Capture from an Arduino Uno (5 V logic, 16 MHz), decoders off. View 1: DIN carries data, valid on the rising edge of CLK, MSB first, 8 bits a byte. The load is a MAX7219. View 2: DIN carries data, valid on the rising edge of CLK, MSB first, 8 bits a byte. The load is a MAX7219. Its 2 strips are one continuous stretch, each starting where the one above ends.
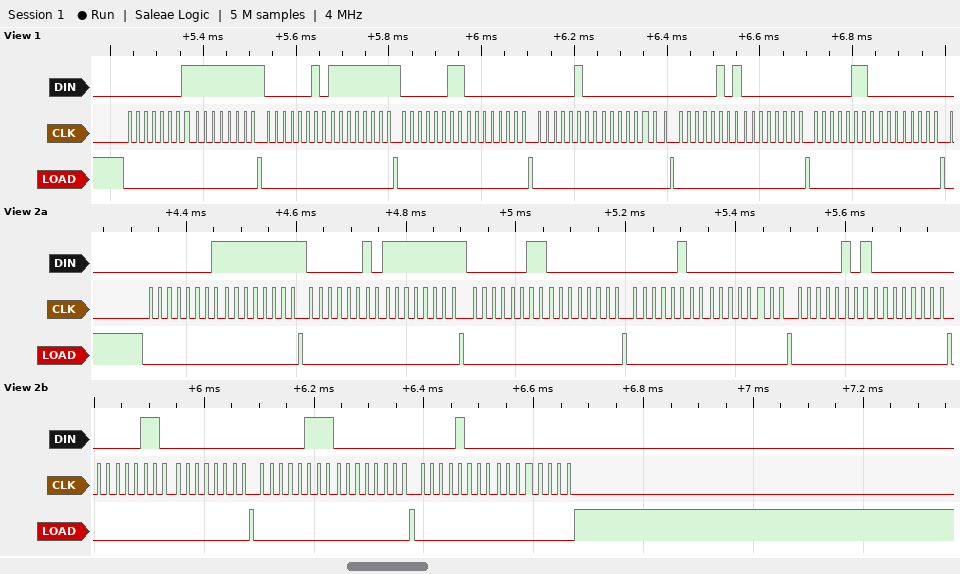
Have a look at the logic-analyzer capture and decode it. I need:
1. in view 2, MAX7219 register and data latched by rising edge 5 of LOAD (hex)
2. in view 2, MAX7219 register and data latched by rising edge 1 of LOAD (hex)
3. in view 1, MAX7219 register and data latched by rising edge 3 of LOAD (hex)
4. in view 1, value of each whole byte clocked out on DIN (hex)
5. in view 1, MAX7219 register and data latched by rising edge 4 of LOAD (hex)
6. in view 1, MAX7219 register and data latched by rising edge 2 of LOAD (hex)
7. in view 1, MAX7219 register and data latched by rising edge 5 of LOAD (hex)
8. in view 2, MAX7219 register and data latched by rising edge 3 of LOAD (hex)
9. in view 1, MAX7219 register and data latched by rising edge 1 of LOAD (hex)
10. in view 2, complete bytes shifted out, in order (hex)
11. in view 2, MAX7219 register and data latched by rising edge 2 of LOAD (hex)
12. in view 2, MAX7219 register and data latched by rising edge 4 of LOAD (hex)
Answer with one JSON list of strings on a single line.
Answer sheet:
["register 0x5, data 0x00", "register 0x1, data 0xFF", "register 0x3, data 0x00", "01 FF 02 FF 03 00 04 00 05 00 06 00", "register 0x4, data 0x00", "register 0x2, data 0xFF", "register 0x5, data 0x00", "register 0x3, data 0x00", "register 0x1, data 0xFF", "01 FF 02 FF 03 00 04 00 05 00 06 00 07 00 08 00", "register 0x2, data 0xFF", "register 0x4, data 0x00"]
